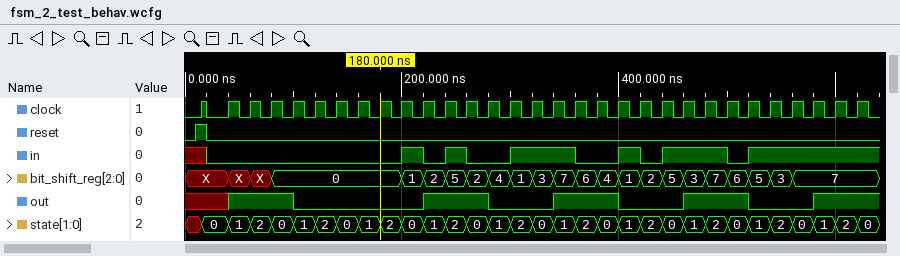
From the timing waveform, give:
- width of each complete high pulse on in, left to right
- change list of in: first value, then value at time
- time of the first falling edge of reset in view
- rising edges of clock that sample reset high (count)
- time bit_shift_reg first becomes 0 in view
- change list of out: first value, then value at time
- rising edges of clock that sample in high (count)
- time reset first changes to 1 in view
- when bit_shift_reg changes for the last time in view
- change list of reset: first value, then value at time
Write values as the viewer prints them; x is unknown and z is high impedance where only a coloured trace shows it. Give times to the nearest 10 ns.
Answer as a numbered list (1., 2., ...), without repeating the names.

1. 20 ns, 20 ns, 60 ns, 20 ns, 60 ns
2. x, 0 at 20 ns, 1 at 200 ns, 0 at 220 ns, 1 at 240 ns, 0 at 260 ns, 1 at 300 ns, 0 at 360 ns, 1 at 400 ns, 0 at 420 ns, 1 at 440 ns, 0 at 500 ns, 1 at 520 ns
3. 20 ns
4. 1
5. 80 ns
6. x, 1 at 40 ns, 0 at 100 ns, 1 at 220 ns, 0 at 280 ns, 1 at 340 ns, 0 at 400 ns, 1 at 460 ns, 0 at 520 ns, 1 at 580 ns
7. 14
8. 10 ns
9. 560 ns
10. 0, 1 at 10 ns, 0 at 20 ns
